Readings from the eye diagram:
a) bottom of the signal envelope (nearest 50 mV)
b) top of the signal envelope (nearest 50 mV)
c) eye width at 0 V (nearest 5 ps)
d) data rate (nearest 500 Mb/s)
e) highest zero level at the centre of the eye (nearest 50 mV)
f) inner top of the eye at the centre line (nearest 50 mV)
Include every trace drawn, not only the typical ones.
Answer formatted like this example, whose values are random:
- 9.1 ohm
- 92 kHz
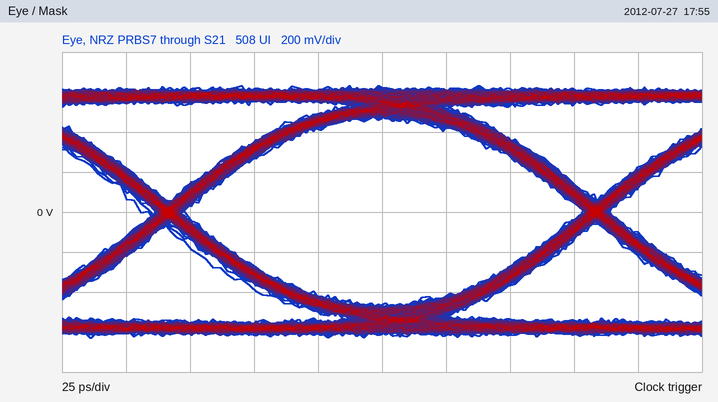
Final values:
- -650 mV
- 650 mV
- 155 ps
- 6.0 Gb/s
- -450 mV
- 450 mV
